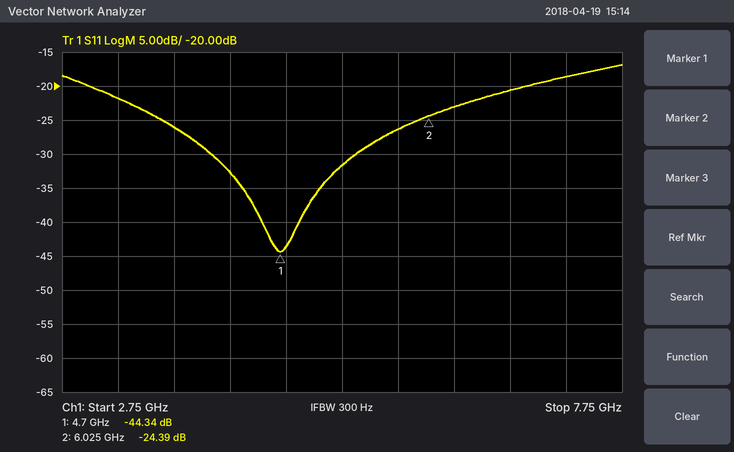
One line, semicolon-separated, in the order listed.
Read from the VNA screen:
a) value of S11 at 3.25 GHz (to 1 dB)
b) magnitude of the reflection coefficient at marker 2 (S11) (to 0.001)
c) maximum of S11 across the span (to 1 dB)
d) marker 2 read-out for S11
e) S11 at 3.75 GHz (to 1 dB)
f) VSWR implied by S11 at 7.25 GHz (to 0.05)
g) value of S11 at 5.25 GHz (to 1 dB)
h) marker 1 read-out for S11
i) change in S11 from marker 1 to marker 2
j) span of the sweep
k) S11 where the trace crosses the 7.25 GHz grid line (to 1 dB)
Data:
-22 dB; 0.060; -17 dB; -24.39 dB; -26 dB; 1.25; -32 dB; -44.34 dB; 19.95 dB; 5 GHz; -19 dB
